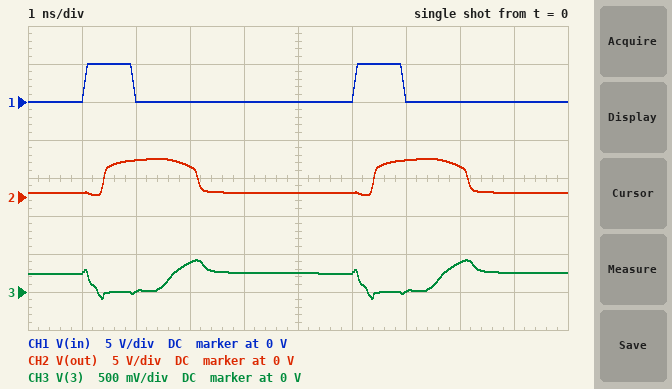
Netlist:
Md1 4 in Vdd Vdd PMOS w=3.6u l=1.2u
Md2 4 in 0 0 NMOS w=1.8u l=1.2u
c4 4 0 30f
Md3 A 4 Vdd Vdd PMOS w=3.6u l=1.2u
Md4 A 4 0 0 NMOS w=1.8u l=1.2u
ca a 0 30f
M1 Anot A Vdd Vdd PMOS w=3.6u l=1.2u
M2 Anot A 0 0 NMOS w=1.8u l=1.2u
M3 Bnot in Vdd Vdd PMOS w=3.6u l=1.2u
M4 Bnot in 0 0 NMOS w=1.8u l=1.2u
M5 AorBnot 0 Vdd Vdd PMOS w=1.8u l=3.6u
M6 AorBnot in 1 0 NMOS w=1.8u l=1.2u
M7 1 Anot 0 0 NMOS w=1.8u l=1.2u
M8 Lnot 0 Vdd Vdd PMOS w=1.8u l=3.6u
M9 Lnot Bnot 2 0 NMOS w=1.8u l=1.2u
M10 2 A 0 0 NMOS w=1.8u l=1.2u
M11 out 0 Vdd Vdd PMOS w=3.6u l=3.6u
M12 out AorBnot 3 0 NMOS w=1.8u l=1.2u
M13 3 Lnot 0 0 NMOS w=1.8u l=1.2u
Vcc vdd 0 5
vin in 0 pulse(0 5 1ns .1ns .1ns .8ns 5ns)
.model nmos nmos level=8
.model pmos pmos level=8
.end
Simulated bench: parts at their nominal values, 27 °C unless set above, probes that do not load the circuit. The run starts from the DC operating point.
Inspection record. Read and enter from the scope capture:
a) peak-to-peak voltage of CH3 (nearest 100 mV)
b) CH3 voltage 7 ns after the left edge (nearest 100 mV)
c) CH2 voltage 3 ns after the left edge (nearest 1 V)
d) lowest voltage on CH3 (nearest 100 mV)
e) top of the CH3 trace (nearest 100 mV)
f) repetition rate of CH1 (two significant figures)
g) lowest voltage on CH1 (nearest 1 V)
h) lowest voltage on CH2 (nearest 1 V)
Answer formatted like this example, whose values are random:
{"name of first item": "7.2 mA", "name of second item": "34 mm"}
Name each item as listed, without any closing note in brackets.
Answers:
{"peak-to-peak voltage of CH3": "500 mV", "CH3 voltage 7 ns after the left edge": "0 V", "CH2 voltage 3 ns after the left edge": "4 V", "lowest voltage on CH3": "-100 mV", "top of the CH3 trace": "400 mV", "repetition rate of CH1": "200 MHz", "lowest voltage on CH1": "0 V", "lowest voltage on CH2": "0 V"}
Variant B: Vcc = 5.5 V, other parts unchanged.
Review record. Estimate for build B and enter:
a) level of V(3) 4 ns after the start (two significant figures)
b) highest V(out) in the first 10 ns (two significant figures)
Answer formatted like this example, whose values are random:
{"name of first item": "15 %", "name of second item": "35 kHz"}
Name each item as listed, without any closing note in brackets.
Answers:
{"level of V(3) 4 ns after the start": "280 mV", "highest V(out) in the first 10 ns": "5.5 V"}
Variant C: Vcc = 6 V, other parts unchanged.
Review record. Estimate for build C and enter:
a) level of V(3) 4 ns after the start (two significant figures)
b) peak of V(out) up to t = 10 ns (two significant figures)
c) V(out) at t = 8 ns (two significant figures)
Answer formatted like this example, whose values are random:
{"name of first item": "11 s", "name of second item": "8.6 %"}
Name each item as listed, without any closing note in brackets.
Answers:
{"level of V(3) 4 ns after the start": "320 mV", "peak of V(out) up to t = 10 ns": "6.0 V", "V(out) at t = 8 ns": "900 mV"}
